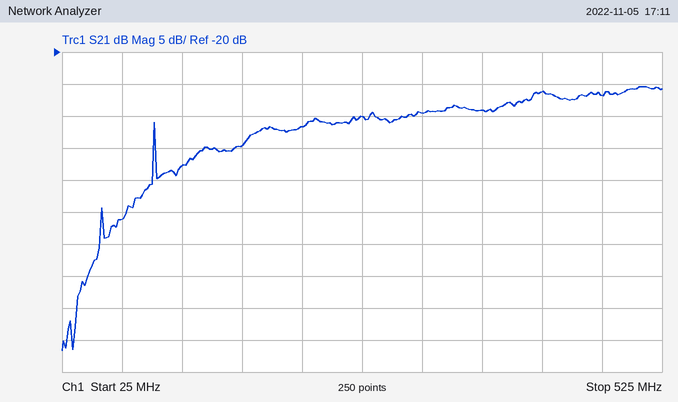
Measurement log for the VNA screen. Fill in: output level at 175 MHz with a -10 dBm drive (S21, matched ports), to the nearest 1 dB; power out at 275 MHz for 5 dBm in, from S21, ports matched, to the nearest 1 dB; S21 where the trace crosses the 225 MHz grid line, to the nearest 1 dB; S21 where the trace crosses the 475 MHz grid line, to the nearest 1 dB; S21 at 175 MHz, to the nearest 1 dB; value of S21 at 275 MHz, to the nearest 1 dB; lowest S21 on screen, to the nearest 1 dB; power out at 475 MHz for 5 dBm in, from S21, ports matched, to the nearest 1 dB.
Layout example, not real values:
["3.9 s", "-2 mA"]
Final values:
["-45 dBm", "-25 dBm", "-32 dB", "-27 dB", "-35 dB", "-30 dB", "-67 dB", "-22 dBm"]
